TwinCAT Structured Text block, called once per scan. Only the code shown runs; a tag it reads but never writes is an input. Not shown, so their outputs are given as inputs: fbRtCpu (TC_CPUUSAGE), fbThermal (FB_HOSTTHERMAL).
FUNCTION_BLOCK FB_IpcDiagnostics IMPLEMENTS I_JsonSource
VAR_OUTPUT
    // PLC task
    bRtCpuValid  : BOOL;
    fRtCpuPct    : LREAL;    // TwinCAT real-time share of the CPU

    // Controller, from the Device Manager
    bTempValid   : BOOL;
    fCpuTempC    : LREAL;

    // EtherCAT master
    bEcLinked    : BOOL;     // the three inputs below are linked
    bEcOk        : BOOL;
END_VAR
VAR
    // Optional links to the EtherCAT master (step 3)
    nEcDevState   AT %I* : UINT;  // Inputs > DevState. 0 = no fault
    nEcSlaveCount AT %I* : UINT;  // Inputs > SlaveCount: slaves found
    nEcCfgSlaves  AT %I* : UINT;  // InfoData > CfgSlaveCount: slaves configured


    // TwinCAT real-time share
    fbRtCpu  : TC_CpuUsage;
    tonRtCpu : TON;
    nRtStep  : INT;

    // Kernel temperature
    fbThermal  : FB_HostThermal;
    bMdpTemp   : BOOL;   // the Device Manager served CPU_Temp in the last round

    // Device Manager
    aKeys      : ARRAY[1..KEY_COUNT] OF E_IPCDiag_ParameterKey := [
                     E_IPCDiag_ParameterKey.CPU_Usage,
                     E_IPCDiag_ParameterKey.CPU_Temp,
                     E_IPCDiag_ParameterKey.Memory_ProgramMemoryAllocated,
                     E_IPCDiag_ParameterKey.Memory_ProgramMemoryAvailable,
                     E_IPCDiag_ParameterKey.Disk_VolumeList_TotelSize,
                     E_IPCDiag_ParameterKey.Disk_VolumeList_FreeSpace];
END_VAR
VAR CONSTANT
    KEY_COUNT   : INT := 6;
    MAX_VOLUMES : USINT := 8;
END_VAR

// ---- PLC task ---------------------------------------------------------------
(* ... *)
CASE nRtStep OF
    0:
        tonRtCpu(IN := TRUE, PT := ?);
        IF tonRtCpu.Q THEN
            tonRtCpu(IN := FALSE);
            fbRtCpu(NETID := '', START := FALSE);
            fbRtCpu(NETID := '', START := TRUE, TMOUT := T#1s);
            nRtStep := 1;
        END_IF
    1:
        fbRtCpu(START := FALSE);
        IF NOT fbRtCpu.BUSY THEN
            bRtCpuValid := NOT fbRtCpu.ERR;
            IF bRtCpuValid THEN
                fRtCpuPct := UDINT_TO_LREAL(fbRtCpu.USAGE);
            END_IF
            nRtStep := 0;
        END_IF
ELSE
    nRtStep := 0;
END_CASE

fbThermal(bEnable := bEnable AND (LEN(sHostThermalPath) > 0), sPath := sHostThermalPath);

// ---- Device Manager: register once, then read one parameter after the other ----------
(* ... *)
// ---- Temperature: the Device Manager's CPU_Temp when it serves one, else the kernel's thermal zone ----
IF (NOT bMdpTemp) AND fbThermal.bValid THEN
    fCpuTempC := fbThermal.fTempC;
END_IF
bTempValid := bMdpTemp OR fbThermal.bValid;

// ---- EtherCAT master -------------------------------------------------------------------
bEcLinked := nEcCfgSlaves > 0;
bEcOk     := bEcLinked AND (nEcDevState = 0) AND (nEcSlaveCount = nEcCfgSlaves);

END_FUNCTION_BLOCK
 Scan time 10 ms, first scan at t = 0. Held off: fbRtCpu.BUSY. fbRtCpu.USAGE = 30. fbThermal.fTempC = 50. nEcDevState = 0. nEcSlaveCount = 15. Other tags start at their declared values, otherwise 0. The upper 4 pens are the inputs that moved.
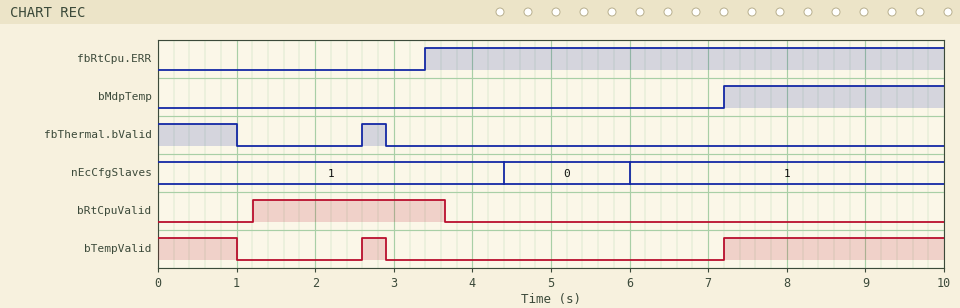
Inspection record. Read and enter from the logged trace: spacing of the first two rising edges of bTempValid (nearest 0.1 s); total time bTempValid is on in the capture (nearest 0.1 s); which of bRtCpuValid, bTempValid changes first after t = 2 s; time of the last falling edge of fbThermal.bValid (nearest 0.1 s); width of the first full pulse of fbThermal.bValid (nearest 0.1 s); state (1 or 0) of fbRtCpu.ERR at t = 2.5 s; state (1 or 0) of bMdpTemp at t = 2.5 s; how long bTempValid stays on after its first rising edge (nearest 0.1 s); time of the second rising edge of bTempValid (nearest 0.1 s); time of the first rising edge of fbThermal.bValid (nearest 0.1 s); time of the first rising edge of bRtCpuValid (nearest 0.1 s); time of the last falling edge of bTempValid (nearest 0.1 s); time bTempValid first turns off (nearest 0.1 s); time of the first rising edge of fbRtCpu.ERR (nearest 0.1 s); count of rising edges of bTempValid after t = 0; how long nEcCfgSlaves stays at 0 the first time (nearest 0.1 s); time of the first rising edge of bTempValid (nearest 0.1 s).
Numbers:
4.6 s
4.1 s
bTempValid
2.9 s
0.3 s
0
0
0.3 s
7.2 s
2.6 s
1.2 s
2.9 s
1.0 s
3.4 s
2
1.6 s
2.6 s
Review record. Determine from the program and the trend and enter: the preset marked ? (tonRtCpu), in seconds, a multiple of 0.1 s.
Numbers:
1.2 s
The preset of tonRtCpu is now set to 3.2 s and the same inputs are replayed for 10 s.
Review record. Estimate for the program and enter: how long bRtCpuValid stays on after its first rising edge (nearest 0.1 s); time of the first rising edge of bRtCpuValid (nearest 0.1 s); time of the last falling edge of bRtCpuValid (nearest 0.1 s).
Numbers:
3.2 s
3.2 s
6.4 s
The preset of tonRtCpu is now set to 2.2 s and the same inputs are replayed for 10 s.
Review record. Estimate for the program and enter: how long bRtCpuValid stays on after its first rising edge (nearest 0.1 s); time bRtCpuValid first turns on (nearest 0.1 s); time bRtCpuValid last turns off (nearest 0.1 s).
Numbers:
2.2 s
2.2 s
4.4 s
